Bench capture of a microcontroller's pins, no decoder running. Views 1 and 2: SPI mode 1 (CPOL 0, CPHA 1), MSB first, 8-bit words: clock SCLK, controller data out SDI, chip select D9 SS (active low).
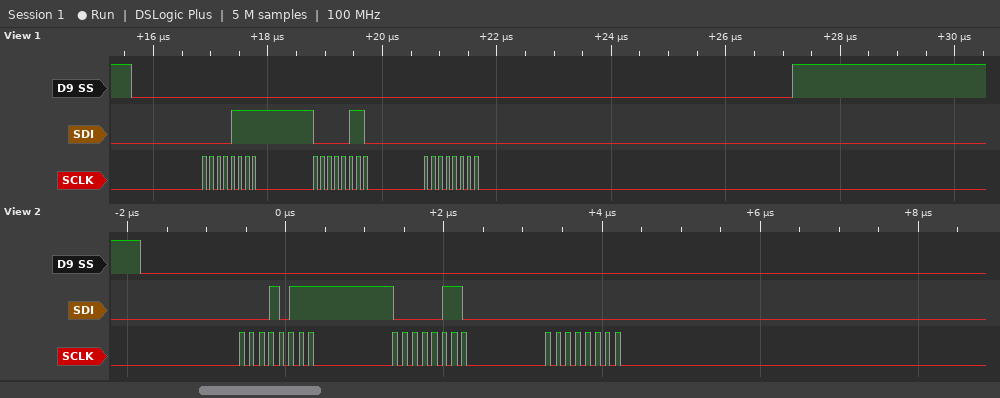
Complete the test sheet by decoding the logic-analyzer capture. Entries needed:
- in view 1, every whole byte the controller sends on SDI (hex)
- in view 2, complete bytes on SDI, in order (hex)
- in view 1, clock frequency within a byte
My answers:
0F 06 00
17 06 00
8 MHz
